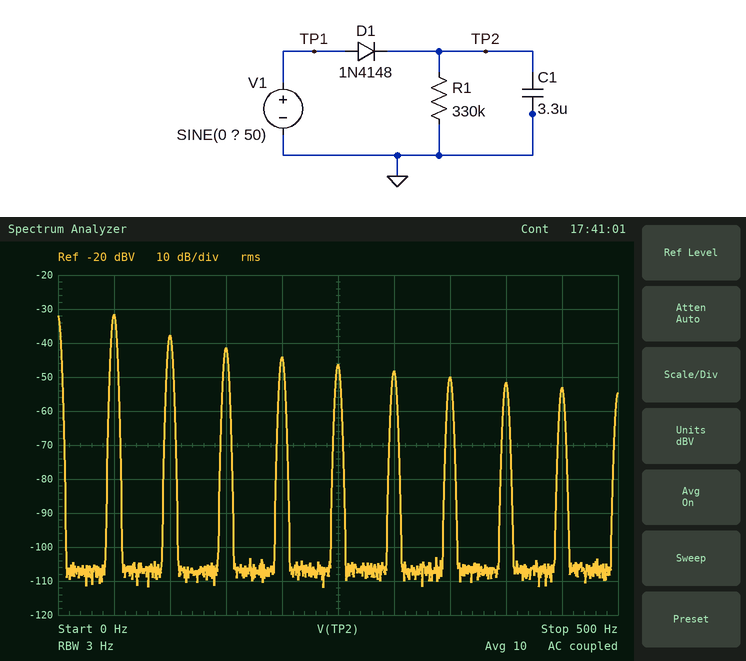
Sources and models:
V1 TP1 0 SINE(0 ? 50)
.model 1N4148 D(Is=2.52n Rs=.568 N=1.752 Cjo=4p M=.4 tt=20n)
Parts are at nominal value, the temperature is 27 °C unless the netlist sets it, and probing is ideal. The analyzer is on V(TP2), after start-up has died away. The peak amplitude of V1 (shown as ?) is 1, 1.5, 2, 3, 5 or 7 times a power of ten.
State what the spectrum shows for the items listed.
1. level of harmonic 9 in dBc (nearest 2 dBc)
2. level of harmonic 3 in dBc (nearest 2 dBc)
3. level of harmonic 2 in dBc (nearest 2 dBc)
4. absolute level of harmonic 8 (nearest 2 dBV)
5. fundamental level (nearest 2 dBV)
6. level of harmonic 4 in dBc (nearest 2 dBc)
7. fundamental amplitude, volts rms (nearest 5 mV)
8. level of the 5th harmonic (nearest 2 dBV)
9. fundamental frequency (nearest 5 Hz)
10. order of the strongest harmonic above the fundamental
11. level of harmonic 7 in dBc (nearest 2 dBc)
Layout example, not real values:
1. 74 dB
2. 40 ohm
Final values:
1. -22 dBc
2. -10 dBc
3. -6 dBc
4. -52 dBV
5. -32 dBV
6. -12 dBc
7. 25 mV
8. -46 dBV
9. 50 Hz
10. 2
11. -18 dBc
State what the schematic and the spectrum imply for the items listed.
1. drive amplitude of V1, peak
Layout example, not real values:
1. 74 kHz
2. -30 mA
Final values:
1. 7 V
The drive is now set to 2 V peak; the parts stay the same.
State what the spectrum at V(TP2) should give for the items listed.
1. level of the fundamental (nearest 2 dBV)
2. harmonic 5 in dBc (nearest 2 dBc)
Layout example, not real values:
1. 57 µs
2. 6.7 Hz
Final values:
1. -44 dBV
2. -16 dBc
